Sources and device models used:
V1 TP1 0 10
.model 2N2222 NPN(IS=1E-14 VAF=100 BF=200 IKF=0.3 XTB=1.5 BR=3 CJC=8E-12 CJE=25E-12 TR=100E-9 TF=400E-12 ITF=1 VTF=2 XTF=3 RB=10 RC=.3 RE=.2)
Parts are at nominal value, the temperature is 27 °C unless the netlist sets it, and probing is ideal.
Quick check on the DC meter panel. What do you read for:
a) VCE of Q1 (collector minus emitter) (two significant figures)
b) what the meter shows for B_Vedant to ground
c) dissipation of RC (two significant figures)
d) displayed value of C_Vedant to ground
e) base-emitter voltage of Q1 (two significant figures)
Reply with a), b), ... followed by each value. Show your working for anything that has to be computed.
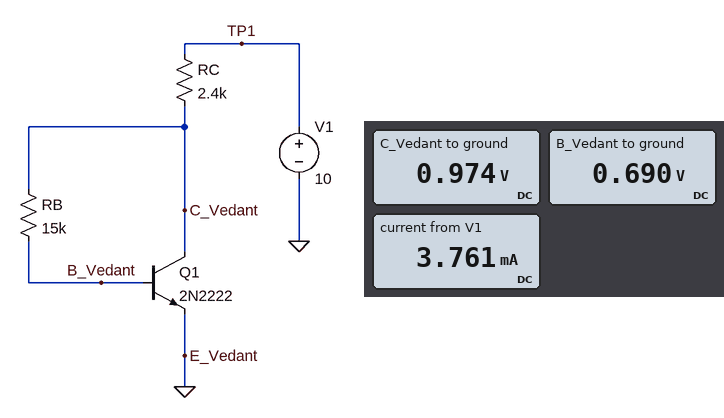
a) 974 mV = 970 mV
b) 0.690 V
c) (10 V - 974 mV)^2 / 2.4 kΩ = 34 mW
d) 0.974 V
e) 690 mV = 690 mV
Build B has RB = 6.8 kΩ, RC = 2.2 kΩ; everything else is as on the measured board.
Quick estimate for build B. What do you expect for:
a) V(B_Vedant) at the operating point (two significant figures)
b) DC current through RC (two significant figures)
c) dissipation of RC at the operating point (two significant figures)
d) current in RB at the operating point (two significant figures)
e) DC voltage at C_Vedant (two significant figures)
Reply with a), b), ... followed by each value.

a) 690 mV
b) 4.2 mA
c) 38 mW
d) 21 µA
e) 840 mV
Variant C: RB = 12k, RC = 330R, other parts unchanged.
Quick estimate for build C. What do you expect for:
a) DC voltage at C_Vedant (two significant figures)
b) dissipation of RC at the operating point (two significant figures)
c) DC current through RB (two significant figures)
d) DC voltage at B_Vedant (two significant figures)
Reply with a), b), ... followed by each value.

a) 2.2 V
b) 180 mW
c) 120 µA
d) 740 mV
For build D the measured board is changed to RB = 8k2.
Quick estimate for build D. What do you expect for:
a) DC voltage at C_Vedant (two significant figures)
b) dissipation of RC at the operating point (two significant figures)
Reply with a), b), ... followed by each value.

a) 850 mV
b) 35 mW
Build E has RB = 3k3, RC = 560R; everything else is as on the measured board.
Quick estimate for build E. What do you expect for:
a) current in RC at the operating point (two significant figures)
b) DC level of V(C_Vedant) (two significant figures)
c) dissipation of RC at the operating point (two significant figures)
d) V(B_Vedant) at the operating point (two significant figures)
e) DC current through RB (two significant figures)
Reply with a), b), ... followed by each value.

a) 16 mA
b) 1.0 V
c) 140 mW
d) 730 mV
e) 84 µA
